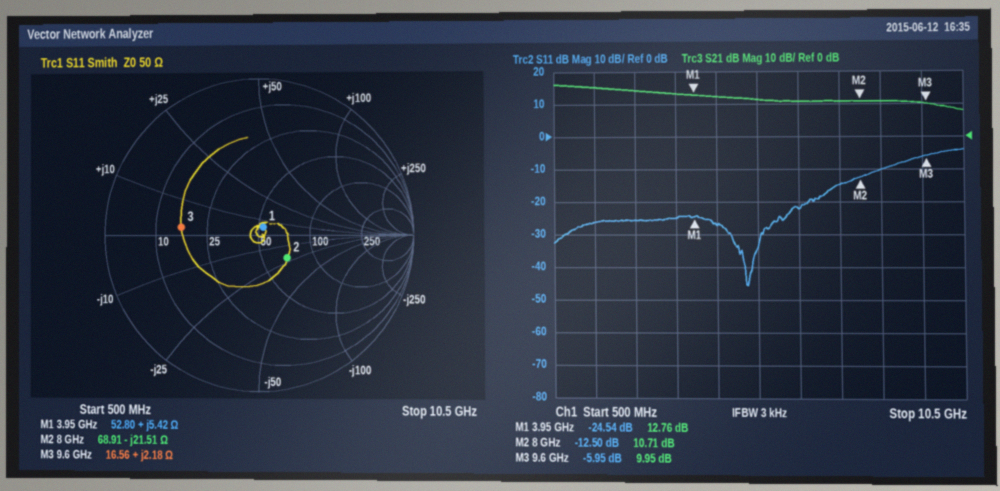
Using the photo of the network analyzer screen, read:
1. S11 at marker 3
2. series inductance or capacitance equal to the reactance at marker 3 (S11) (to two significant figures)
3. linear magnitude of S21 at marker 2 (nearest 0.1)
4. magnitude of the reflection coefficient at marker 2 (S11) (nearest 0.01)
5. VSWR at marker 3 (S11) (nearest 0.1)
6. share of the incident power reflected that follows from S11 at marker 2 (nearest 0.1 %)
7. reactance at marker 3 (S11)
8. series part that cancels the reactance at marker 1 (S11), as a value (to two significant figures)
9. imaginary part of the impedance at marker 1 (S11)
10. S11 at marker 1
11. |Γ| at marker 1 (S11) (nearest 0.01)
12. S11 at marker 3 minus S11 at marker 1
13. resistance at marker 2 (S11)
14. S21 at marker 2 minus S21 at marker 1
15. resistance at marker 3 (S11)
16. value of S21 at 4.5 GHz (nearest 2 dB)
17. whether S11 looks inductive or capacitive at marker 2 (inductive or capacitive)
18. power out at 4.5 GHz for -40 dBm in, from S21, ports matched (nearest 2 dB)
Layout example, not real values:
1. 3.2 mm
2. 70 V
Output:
1. -5.95 dB
2. 36 pH
3. 3.4
4. 0.24
5. 3.0
6. 5.6 %
7. +2.18 Ω
8. 7.4 pF
9. +5.42 Ω
10. -24.54 dB
11. 0.06
12. 18.59 dB
13. 68.91 Ω
14. -2.05 dB
15. 16.56 Ω
16. 12 dB
17. capacitive
18. -28 dBm
